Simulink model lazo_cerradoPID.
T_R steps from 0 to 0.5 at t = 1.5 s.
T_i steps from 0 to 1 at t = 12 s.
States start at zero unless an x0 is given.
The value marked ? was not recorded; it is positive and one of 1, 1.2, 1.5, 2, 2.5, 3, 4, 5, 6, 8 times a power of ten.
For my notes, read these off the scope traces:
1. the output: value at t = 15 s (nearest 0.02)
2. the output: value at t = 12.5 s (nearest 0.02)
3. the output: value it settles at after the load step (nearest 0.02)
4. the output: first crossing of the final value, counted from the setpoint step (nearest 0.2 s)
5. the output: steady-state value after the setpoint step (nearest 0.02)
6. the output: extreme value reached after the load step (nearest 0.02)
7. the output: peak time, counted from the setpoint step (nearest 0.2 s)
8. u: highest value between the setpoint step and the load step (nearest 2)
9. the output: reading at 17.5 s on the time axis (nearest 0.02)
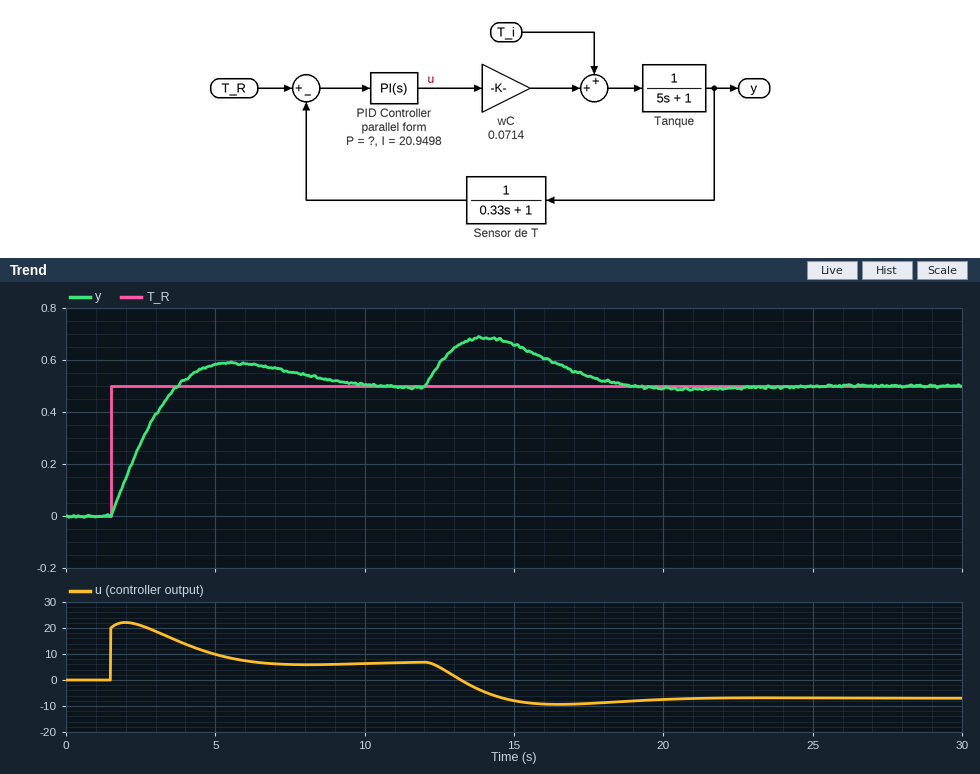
0.66
0.58
0.50
2.2 s
0.50
0.68
4.0 s
22
0.54
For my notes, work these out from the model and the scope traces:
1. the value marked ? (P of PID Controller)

40
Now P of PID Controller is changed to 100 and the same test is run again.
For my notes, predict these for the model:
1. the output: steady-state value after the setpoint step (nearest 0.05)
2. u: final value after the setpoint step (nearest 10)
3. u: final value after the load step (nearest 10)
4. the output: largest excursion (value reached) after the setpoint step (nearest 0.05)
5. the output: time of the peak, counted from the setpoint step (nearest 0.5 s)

0.50
10
-10
0.55
1.5 s
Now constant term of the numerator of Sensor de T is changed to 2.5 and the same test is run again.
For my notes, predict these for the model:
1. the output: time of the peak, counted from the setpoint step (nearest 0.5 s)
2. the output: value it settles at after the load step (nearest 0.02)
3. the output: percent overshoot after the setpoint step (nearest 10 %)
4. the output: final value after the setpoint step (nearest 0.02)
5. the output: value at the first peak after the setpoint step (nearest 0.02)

1.5 s
0.20
20 %
0.20
0.24
